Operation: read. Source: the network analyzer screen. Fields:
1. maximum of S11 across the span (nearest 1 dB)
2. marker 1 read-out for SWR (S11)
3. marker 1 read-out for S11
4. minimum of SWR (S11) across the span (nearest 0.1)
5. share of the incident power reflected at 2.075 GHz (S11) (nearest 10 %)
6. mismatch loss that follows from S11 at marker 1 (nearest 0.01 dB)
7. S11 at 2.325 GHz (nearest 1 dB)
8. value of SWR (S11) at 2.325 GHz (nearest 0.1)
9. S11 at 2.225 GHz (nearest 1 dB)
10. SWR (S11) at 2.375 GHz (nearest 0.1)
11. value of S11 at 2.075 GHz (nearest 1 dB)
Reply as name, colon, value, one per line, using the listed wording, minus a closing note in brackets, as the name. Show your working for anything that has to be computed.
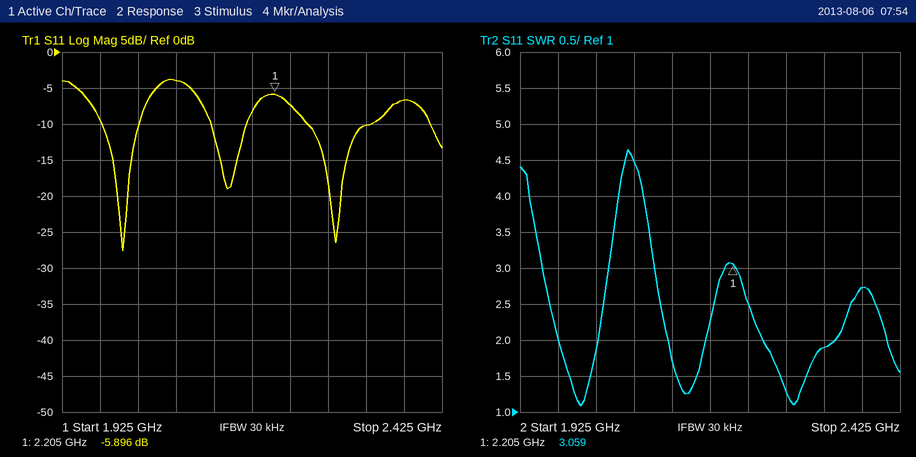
maximum of S11 across the span: -4 dB
marker 1 read-out for SWR: 3.059
marker 1 read-out for S11: -5.896 dB
minimum of SWR (S11) across the span: 1.1
share of the incident power reflected at 2.075 GHz (S11): 10^(-4/10) ≈ 40 %
mismatch loss that follows from S11 at marker 1: −10 log10(1 − 10^(-5.896/10)) ≈ 1.29 dB
S11 at 2.325 GHz: -10 dB
value of SWR (S11) at 2.325 GHz: 1.9
S11 at 2.225 GHz: -7 dB
SWR (S11) at 2.375 GHz: 2.7
value of S11 at 2.075 GHz: -4 dB
